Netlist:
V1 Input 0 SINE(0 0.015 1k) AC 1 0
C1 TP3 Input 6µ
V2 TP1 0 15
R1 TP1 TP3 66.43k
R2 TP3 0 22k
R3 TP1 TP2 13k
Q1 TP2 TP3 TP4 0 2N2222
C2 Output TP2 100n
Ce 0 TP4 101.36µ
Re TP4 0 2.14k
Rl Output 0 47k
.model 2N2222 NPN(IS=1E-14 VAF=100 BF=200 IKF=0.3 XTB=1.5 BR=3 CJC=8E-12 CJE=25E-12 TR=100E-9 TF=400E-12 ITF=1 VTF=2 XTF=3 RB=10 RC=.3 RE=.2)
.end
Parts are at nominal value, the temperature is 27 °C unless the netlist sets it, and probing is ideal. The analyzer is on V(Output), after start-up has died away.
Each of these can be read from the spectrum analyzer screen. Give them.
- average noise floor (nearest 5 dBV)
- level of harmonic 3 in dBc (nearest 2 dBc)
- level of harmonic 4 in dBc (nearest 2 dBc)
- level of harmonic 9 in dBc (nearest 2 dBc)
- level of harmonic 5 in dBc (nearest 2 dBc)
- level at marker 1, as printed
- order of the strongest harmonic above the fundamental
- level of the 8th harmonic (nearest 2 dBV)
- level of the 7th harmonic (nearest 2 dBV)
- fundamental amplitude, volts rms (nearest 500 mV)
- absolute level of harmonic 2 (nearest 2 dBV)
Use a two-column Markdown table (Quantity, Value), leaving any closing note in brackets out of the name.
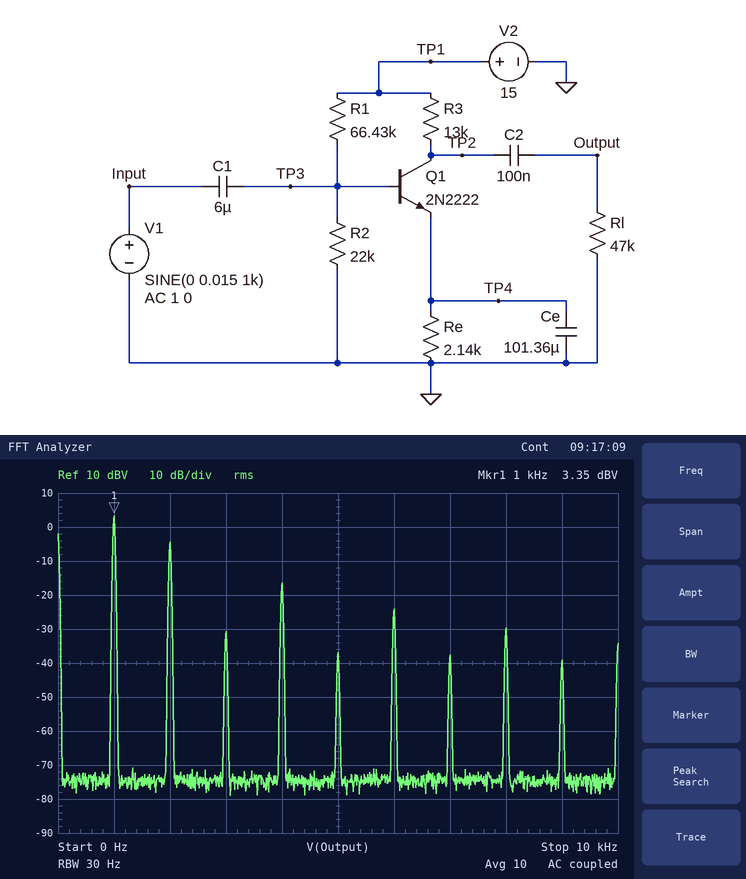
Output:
| Quantity | Value |
|---|---|
| average noise floor | -75 dBV |
| level of harmonic 3 in dBc | -34 dBc |
| level of harmonic 4 in dBc | -20 dBc |
| level of harmonic 9 in dBc | -42 dBc |
| level of harmonic 5 in dBc | -40 dBc |
| level at marker 1, as printed | 3.35 dBV |
| order of the strongest harmonic above the fundamental | 2 |
| level of the 8th harmonic | -30 dBV |
| level of the 7th harmonic | -38 dBV |
| fundamental amplitude, volts rms | 1.5 V |
| absolute level of harmonic 2 | -4 dBV |
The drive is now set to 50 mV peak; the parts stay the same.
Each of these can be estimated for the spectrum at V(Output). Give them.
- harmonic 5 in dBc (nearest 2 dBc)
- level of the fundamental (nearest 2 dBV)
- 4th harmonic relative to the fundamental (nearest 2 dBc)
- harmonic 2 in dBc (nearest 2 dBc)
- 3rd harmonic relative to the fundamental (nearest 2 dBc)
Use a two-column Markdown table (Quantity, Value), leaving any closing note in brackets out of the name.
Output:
| Quantity | Value |
|---|---|
| harmonic 5 in dBc | -30 dBc |
| level of the fundamental | 12 dBV |
| 4th harmonic relative to the fundamental | -22 dBc |
| harmonic 2 in dBc | -26 dBc |
| 3rd harmonic relative to the fundamental | -14 dBc |
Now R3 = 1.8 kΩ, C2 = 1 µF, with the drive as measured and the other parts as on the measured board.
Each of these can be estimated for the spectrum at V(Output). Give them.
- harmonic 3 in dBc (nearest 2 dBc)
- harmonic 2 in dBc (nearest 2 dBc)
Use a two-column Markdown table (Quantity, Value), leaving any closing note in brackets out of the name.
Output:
| Quantity | Value |
|---|---|
| harmonic 3 in dBc | -40 dBc |
| harmonic 2 in dBc | -18 dBc |
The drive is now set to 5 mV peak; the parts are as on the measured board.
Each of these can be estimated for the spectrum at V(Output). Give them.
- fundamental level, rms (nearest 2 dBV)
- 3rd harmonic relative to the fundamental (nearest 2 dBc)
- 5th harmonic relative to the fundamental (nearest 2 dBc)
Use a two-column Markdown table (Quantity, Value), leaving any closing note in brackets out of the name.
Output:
| Quantity | Value |
|---|---|
| fundamental level, rms | -32 dBV |
| 3rd harmonic relative to the fundamental | -14 dBc |
| 5th harmonic relative to the fundamental | -24 dBc |
